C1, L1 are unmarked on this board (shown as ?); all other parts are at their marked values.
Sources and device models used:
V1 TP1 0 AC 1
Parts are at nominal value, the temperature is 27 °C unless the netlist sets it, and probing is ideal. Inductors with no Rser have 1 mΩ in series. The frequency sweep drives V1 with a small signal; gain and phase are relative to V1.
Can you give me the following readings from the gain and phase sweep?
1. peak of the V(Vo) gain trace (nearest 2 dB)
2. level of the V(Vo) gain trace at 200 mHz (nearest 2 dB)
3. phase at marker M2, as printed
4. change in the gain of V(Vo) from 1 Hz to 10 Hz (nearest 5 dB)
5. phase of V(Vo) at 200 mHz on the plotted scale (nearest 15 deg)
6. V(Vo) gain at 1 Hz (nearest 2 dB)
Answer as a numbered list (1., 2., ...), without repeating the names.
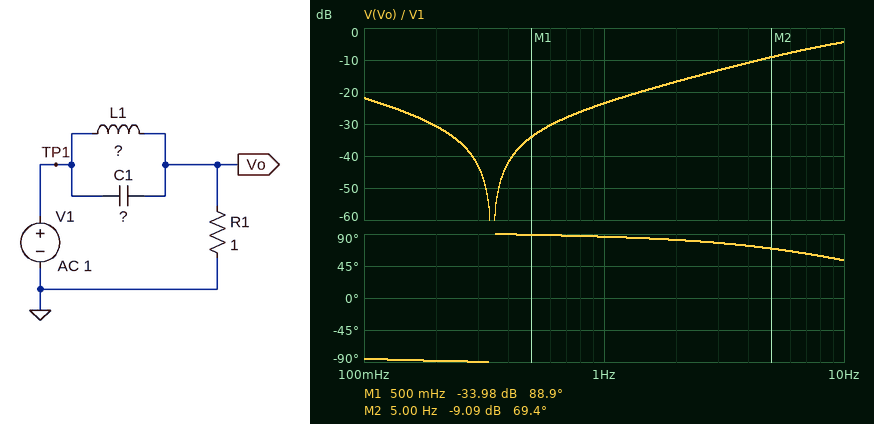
1. -4 dB
2. -30 dB
3. 69.4 deg
4. 20 dB
5. -90 deg
6. -24 dB
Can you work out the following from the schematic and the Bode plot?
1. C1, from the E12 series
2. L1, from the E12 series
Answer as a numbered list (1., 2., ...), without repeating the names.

1. 12 mF
2. 18 H
